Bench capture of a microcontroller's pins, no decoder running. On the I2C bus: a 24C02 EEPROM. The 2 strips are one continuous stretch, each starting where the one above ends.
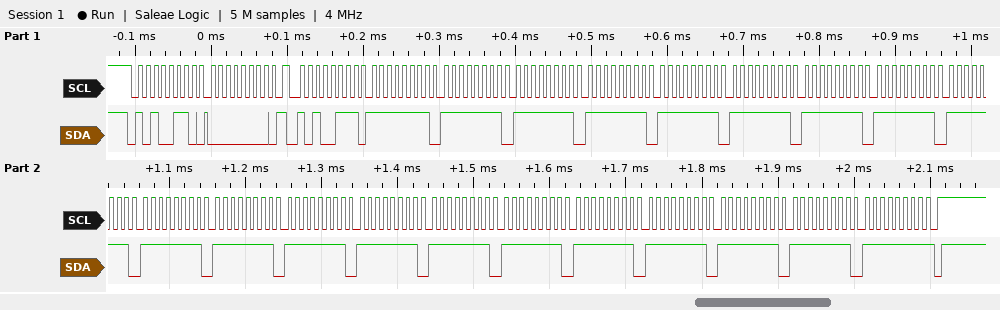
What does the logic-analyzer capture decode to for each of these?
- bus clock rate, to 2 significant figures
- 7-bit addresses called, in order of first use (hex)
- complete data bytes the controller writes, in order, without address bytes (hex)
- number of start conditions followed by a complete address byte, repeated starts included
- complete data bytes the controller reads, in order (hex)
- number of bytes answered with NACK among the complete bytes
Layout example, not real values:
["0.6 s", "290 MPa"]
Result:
["100 kHz", "0x53", "00", "2", "FF FF FF FF FF FF FF FF FF FF FF FF FF FF FF FF FF FF FF FF", "1"]
